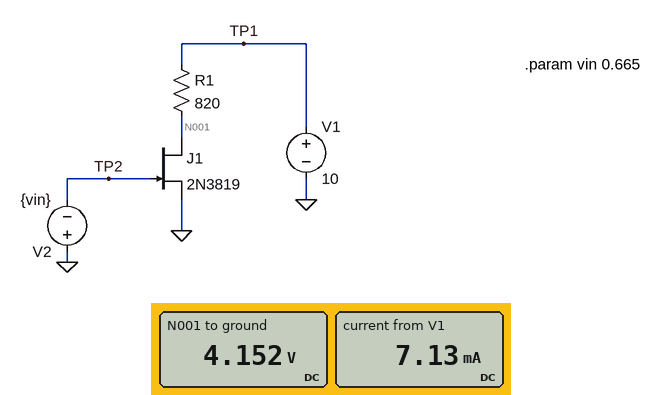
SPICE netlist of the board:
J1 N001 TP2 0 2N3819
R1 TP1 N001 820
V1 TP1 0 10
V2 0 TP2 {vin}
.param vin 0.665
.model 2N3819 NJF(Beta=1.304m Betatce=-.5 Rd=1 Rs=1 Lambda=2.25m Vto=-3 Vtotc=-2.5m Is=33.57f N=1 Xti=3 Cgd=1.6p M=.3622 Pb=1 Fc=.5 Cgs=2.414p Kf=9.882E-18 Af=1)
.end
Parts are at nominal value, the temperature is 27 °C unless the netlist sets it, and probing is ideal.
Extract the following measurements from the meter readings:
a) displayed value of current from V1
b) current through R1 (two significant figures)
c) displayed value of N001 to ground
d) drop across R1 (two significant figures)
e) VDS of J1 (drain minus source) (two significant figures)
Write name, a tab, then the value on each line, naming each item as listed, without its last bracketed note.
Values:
displayed value of current from V1	7.13 mA
current through R1	7.1 mA
displayed value of N001 to ground	4.152 V
drop across R1	5.8 V
VDS of J1 (drain minus source)	4.2 V
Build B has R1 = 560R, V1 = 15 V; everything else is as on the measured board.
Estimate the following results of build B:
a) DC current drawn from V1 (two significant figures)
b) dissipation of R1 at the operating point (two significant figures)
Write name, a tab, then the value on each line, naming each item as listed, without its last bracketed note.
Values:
DC current drawn from V1	7.2 mA
dissipation of R1 at the operating point	29 mW
